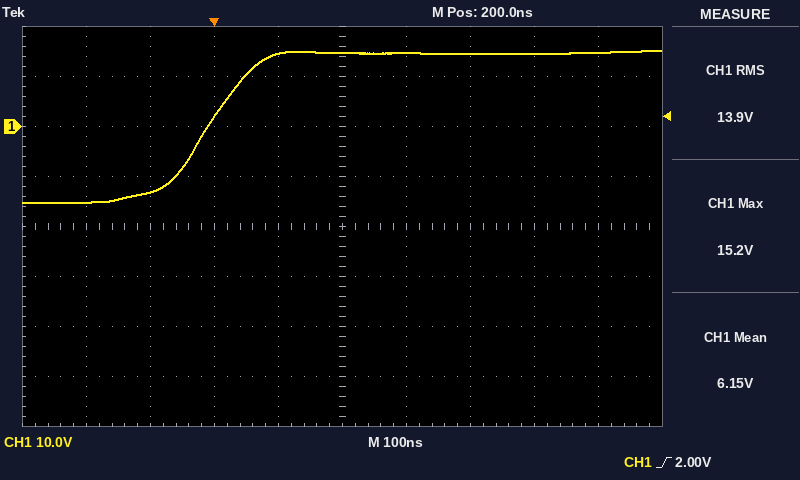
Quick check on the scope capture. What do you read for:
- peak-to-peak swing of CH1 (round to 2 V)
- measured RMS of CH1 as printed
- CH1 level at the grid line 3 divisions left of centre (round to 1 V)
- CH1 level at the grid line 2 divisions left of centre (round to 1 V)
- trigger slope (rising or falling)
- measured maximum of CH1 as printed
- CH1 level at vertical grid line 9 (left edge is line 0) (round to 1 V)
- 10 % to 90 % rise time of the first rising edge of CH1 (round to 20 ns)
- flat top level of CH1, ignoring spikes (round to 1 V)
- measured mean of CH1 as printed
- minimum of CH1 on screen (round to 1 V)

30 V
13.9 V
-13 V
2 V
rising
15.2 V
15 V
140 ns
15 V
6.15 V
-15 V
